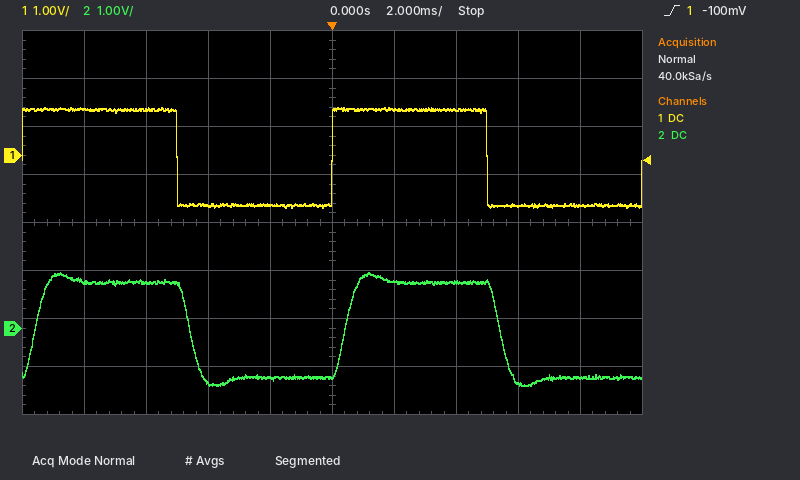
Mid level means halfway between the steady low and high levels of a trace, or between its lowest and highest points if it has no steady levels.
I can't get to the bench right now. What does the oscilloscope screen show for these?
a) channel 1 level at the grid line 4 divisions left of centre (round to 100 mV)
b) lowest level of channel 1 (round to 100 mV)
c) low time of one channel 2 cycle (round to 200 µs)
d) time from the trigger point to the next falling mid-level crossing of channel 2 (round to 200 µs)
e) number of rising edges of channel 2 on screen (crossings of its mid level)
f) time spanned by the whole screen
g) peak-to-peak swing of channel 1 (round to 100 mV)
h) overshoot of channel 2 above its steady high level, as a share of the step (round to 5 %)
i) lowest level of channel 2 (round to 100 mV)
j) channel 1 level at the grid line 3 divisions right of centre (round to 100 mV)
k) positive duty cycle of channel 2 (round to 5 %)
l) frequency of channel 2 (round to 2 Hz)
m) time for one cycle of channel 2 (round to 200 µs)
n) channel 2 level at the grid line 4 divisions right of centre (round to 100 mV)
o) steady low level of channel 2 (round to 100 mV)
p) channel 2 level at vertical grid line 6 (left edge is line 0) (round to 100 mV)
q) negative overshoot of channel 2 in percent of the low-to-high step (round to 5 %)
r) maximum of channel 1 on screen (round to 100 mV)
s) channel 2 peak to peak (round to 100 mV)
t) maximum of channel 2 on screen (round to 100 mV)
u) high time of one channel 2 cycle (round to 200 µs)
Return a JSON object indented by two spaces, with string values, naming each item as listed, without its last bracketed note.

{
  "channel 1 level at the grid line 4 divisions left of centre": "1.0 V",
  "lowest level of channel 1": "-1.1 V",
  "low time of one channel 2 cycle": "5.0 ms",
  "time from the trigger point to the next falling mid-level crossing of channel 2": "5.4 ms",
  "number of rising edges of channel 2 on screen": "2",
  "time spanned by the whole screen": "20 ms",
  "peak-to-peak swing of channel 1": "2.1 V",
  "overshoot of channel 2 above its steady high level, as a share of the step": "10 %",
  "lowest level of channel 2": "-1.2 V",
  "channel 1 level at the grid line 3 divisions right of centre": "-1.1 V",
  "positive duty cycle of channel 2": "50 %",
  "frequency of channel 2": "100 Hz",
  "time for one cycle of channel 2": "10.0 ms",
  "channel 2 level at the grid line 4 divisions right of centre": "-1.0 V",
  "steady low level of channel 2": "-1.0 V",
  "channel 2 level at vertical grid line 6 (left edge is line 0)": "1.0 V",
  "negative overshoot of channel 2 in percent of the low-to-high step": "10 %",
  "maximum of channel 1 on screen": "1.0 V",
  "channel 2 peak to peak": "2.4 V",
  "maximum of channel 2 on screen": "1.2 V",
  "high time of one channel 2 cycle": "5.0 ms"
}
